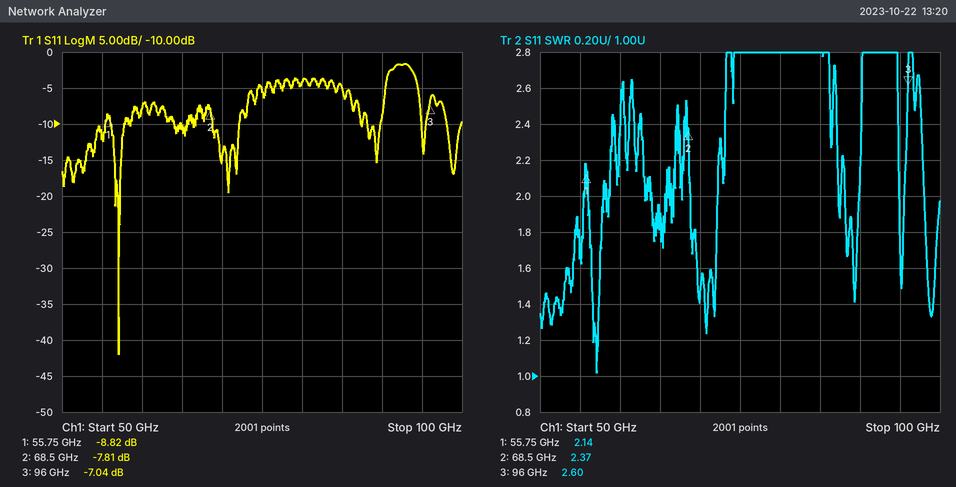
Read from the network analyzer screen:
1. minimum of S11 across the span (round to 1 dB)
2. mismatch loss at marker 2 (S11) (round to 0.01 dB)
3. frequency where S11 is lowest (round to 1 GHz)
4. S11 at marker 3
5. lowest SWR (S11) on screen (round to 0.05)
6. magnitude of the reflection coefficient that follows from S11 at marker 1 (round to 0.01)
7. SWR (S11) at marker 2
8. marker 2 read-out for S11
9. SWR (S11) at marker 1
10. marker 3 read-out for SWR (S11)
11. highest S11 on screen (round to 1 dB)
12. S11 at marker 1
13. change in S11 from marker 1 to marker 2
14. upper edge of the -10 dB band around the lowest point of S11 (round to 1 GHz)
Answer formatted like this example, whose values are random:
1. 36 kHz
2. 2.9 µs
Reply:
1. -42 dB
2. 0.79 dB
3. 57 GHz
4. -7.04 dB
5. 1.00
6. 0.36
7. 2.37
8. -7.81 dB
9. 2.14
10. 2.60
11. -2 dB
12. -8.82 dB
13. 1.01 dB
14. 58 GHz
